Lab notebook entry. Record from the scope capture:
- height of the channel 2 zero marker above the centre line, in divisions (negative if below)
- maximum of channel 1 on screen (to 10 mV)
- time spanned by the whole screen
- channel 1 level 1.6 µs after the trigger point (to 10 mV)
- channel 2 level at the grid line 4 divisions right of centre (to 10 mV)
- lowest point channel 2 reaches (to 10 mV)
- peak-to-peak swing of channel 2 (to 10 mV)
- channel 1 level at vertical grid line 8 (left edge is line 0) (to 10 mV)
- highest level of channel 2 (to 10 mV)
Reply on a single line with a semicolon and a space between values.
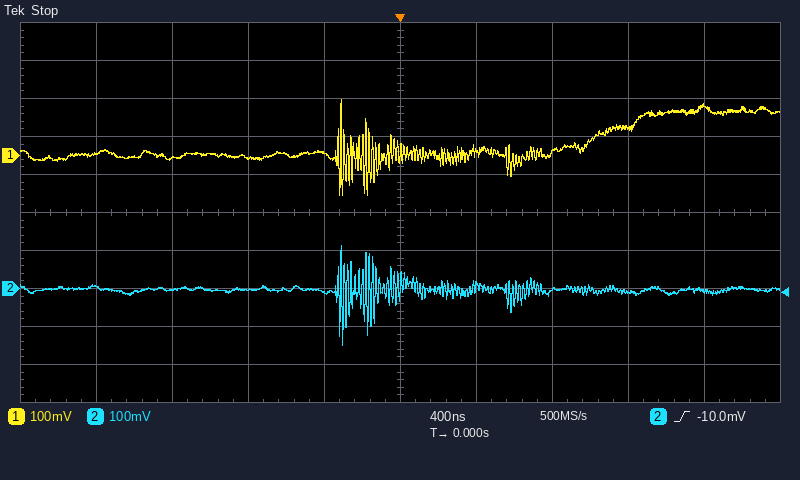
-2.0 div; 150 mV; 4 µs; 130 mV; -10 mV; -150 mV; 260 mV; 70 mV; 110 mV
